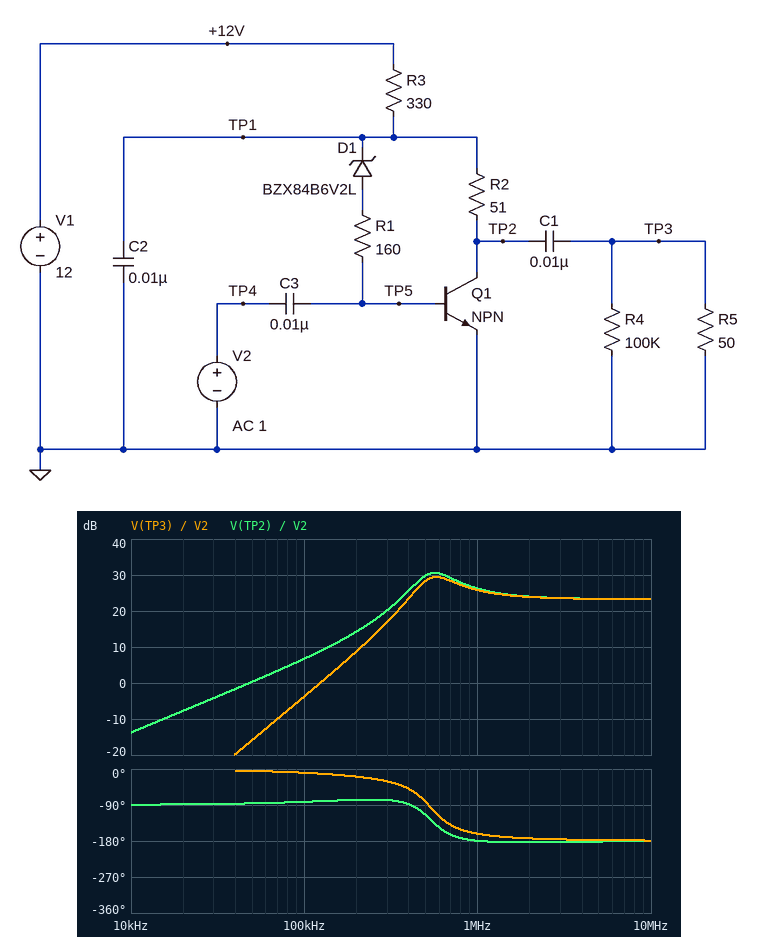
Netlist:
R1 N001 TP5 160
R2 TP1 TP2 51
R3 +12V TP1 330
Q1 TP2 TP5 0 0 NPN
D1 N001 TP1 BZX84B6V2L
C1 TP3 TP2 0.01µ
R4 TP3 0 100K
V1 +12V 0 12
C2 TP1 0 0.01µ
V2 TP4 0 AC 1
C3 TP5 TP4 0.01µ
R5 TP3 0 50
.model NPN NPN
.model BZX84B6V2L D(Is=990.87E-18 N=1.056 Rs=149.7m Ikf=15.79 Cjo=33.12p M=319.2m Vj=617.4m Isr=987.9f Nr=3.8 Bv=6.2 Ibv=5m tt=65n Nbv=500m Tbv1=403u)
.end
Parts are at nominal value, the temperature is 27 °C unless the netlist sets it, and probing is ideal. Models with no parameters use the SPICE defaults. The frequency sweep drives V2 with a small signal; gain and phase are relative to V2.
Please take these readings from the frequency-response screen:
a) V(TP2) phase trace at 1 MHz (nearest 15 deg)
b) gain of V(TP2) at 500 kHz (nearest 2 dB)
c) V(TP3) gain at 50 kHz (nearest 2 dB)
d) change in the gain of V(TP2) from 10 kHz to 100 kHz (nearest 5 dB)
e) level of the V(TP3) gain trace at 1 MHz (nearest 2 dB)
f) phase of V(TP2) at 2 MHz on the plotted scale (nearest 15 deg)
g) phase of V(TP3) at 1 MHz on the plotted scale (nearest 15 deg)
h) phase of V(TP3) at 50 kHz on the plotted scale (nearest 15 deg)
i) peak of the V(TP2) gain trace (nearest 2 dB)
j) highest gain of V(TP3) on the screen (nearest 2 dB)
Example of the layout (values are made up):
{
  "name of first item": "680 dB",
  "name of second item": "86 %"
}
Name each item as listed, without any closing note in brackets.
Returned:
{
  "V(TP2) phase trace at 1 MHz": "-180 deg",
  "gain of V(TP2) at 500 kHz": "30 dB",
  "V(TP3) gain at 50 kHz": "-16 dB",
  "change in the gain of V(TP2) from 10 kHz to 100 kHz": "20 dB",
  "level of the V(TP3) gain trace at 1 MHz": "26 dB",
  "phase of V(TP2) at 2 MHz on the plotted scale": "-180 deg",
  "phase of V(TP3) at 1 MHz on the plotted scale": "-165 deg",
  "phase of V(TP3) at 50 kHz on the plotted scale": "0 deg",
  "peak of the V(TP2) gain trace": "30 dB",
  "highest gain of V(TP3) on the screen": "30 dB"
}
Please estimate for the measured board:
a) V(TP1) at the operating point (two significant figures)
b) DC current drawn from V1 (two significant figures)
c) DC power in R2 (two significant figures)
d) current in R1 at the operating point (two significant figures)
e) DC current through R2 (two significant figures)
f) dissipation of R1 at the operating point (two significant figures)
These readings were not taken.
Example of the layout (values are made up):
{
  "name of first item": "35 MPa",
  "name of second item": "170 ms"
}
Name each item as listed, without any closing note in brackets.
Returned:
{
  "V(TP1) at the operating point": "7.0 V",
  "DC current drawn from V1": "15 mA",
  "DC power in R2": "11 mW",
  "current in R1 at the operating point": "150 µA",
  "DC current through R2": "15 mA",
  "dissipation of R1 at the operating point": "3.6 µW"
}
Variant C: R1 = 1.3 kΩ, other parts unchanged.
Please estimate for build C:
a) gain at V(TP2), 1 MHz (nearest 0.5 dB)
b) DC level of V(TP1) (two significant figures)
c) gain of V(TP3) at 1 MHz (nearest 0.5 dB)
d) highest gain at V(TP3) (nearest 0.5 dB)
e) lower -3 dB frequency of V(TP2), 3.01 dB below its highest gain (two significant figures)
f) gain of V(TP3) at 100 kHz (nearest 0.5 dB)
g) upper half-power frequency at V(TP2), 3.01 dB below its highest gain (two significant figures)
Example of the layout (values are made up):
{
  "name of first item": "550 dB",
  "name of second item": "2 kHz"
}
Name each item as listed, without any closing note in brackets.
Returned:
{
  "gain at V(TP2), 1 MHz": "24.0 dB",
  "DC level of V(TP1)": "7.2 V",
  "gain of V(TP3) at 1 MHz": "23.5 dB",
  "highest gain at V(TP3)": "28.0 dB",
  "lower -3 dB frequency of V(TP2), 3.01 dB below its highest gain": "170 kHz",
  "gain of V(TP3) at 100 kHz": "11.0 dB",
  "upper half-power frequency at V(TP2), 3.01 dB below its highest gain": "330 kHz"
}
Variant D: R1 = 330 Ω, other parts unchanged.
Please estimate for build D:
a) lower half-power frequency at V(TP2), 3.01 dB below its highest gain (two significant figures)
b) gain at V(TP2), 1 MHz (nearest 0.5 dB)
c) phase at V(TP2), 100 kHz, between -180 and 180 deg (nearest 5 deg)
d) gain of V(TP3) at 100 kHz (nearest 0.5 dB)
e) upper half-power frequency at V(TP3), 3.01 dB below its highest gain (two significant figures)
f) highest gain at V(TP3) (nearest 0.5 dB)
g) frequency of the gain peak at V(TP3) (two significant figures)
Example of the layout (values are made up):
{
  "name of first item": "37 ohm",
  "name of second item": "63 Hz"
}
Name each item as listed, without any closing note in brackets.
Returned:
{
  "lower half-power frequency at V(TP2), 3.01 dB below its highest gain": "340 kHz",
  "gain at V(TP2), 1 MHz": "25.0 dB",
  "phase at V(TP2), 100 kHz, between -180 and 180 deg": "-85 deg",
  "gain of V(TP3) at 100 kHz": "0.5 dB",
  "upper half-power frequency at V(TP3), 3.01 dB below its highest gain": "660 kHz",
  "highest gain at V(TP3)": "30.0 dB",
  "frequency of the gain peak at V(TP3)": "440 kHz"
}
